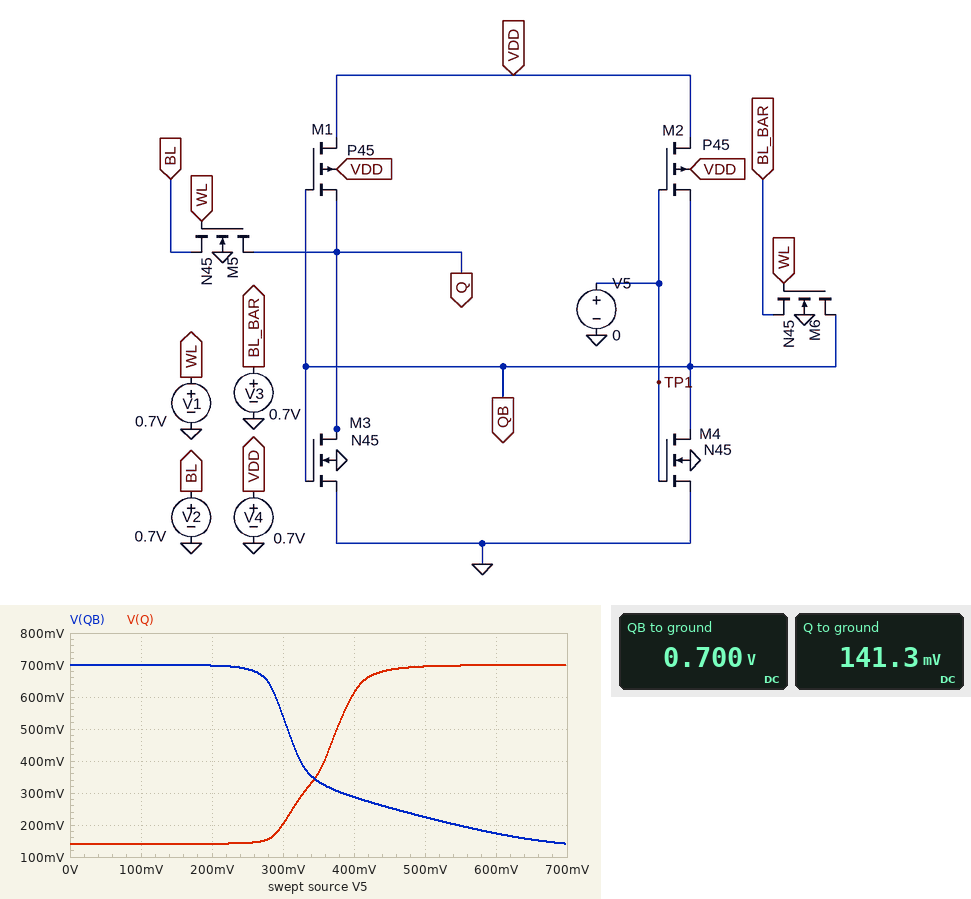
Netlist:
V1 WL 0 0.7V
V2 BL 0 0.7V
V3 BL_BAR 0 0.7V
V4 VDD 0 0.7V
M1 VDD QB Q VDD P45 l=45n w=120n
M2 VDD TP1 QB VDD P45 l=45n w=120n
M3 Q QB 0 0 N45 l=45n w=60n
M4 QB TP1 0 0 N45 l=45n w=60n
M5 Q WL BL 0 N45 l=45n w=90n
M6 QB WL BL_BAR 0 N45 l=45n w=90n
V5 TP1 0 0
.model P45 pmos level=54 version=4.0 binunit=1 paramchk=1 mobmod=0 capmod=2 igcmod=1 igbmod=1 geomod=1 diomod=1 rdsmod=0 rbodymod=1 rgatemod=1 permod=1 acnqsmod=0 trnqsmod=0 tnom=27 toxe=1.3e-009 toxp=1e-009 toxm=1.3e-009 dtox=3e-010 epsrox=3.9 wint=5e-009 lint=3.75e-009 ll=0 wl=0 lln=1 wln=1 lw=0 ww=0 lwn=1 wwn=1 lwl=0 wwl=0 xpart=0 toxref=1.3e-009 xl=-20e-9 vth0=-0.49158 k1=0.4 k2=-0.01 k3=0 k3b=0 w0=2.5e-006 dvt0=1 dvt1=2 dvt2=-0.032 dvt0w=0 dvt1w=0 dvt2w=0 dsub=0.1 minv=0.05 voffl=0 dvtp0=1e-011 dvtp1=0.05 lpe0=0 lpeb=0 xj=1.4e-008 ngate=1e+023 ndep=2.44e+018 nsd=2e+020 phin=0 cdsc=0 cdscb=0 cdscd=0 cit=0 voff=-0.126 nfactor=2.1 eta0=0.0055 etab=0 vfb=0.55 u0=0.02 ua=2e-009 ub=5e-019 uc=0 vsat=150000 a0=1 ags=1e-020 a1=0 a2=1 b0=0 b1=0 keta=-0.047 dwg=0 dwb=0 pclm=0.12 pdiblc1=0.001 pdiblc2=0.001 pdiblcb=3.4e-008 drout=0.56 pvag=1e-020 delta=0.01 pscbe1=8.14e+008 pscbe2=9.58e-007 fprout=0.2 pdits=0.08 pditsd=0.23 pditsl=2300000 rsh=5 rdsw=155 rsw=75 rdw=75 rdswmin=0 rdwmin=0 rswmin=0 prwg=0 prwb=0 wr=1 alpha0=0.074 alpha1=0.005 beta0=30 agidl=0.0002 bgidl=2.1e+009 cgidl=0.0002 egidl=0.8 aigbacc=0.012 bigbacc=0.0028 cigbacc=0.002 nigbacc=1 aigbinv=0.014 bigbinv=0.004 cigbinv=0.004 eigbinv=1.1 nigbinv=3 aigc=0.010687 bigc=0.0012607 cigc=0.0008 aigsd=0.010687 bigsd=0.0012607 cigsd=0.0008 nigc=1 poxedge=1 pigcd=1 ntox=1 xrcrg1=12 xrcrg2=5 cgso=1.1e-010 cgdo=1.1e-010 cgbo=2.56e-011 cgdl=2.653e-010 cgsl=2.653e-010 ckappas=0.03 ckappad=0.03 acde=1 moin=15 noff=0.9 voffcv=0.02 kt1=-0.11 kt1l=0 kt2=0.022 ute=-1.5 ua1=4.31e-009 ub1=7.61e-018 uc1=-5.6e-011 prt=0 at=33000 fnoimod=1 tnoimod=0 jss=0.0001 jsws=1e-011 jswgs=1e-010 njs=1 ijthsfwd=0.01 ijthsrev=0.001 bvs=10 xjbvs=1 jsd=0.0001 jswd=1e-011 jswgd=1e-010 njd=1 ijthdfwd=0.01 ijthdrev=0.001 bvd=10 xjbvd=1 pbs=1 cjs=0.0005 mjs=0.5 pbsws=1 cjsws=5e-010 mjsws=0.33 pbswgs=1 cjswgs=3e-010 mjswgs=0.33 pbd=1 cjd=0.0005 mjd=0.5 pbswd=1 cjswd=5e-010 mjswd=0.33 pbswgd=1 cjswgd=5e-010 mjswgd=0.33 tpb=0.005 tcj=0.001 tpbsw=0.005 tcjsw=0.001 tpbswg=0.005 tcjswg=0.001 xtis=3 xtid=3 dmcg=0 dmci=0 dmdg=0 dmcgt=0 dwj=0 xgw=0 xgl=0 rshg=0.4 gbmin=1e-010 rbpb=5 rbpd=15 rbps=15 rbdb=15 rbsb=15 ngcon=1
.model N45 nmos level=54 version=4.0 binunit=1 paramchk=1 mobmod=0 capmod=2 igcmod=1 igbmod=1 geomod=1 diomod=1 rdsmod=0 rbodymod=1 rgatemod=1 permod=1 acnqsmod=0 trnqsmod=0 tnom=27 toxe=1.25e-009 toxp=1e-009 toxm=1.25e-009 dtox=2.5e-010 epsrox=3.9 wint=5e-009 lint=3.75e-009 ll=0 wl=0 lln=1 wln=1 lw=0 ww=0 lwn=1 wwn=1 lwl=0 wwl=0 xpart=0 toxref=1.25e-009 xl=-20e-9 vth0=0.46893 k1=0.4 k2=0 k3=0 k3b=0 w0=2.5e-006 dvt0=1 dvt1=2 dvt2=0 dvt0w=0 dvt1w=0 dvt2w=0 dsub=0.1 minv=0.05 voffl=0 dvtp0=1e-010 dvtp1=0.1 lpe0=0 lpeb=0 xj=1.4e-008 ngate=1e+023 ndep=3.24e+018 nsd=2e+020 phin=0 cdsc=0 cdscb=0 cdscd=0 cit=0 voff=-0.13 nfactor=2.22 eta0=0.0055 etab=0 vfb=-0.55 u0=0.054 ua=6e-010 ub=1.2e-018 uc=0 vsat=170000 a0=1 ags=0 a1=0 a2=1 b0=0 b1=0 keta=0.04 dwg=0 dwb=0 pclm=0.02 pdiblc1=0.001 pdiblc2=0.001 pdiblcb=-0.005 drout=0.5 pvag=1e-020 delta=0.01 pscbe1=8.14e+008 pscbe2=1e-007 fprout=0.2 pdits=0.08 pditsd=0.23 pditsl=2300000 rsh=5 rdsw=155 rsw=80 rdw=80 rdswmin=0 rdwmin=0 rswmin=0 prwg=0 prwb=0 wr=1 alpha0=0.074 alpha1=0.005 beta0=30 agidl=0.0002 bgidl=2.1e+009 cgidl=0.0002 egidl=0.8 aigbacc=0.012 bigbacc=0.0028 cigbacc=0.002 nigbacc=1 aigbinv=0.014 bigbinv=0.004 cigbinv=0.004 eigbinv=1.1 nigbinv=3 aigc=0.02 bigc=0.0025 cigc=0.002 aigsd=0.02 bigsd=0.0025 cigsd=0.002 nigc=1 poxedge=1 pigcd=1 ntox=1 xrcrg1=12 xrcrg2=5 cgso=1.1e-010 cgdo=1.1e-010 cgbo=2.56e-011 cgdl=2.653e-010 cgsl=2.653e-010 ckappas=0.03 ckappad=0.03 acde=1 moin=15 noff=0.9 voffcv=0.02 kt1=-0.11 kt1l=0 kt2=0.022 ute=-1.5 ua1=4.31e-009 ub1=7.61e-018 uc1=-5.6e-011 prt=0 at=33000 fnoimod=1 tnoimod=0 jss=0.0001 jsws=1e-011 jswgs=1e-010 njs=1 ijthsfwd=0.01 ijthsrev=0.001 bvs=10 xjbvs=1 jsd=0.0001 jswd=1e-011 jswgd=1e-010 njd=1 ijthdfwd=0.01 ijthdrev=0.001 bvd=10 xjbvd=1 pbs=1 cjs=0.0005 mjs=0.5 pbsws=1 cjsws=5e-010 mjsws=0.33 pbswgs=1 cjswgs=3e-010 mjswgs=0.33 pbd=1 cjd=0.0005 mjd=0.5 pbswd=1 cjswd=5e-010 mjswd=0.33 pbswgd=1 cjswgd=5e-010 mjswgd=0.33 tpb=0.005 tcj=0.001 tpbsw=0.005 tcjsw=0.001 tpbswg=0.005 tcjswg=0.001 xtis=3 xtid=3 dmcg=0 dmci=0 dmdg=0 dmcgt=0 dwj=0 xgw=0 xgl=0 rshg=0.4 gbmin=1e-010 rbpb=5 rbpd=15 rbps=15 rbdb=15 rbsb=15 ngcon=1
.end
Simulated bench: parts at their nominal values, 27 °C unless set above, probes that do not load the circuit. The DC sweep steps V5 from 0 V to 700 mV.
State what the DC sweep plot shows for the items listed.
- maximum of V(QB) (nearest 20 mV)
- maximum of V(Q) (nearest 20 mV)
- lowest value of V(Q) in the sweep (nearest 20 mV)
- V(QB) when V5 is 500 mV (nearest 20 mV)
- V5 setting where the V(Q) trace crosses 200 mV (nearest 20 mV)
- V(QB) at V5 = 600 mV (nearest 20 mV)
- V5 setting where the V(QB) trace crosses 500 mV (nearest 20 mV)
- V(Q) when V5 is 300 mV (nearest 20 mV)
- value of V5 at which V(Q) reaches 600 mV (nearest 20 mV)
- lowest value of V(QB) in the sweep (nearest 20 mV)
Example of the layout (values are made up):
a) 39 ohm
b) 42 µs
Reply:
a) 700 mV
b) 700 mV
c) 140 mV
d) 220 mV
e) 300 mV
f) 180 mV
g) 300 mV
h) 200 mV
i) 400 mV
j) 140 mV
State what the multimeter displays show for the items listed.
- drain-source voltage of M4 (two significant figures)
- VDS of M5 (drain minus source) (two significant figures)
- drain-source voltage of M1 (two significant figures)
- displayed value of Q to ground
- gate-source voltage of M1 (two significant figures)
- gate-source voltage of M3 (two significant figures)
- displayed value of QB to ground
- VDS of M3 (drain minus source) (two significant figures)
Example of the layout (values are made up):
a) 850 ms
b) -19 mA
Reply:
a) 700 mV
b) -560 mV
c) 560 mV
d) 141.3 mV
e) 560 mV
f) 700 mV
g) 0.700 V
h) 140 mV
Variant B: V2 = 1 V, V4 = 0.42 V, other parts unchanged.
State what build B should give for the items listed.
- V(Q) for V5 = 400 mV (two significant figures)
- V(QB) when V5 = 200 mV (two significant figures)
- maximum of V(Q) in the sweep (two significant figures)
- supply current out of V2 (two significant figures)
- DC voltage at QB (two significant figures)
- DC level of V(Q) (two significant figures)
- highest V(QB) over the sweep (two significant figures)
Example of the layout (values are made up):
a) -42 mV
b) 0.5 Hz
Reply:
a) 390 mV
b) 410 mV
c) 450 mV
d) 1.9 µA
e) 420 mV
f) 300 mV
g) 430 mV
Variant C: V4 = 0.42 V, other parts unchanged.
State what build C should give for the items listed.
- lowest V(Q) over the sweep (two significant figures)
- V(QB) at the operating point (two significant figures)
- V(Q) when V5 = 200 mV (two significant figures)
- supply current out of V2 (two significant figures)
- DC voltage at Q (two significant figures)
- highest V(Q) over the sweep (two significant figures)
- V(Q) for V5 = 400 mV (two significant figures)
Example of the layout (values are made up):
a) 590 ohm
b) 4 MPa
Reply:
a) 260 mV
b) 420 mV
c) 280 mV
d) 1.8 µA
e) 270 mV
f) 430 mV
g) 360 mV
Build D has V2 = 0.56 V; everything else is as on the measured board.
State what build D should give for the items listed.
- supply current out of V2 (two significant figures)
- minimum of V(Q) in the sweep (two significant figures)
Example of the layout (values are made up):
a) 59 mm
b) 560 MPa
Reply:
a) 17 µA
b) 130 mV
